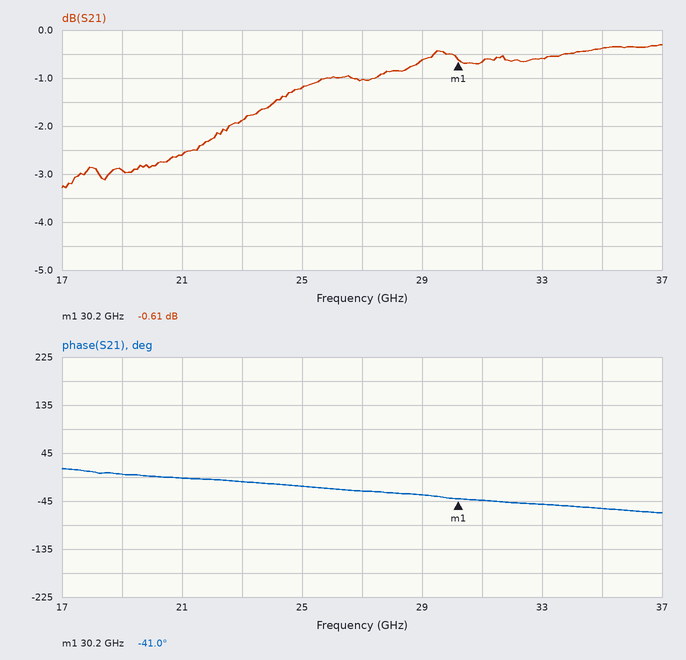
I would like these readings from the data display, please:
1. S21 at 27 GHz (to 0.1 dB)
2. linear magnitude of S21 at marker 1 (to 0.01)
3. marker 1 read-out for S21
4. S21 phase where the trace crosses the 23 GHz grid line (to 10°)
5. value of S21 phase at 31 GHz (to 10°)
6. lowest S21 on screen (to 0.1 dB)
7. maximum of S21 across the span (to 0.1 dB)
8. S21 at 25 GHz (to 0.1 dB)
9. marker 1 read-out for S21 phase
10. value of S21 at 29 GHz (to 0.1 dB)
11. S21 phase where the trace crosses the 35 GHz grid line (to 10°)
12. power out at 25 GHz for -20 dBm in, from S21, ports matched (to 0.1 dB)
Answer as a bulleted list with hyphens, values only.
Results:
- -1.0 dB
- 0.93
- -0.61 dB
- -10°
- -40°
- -3.3 dB
- -0.3 dB
- -1.2 dB
- -41.0°
- -0.6 dB
- -60°
- -21.2 dBm
